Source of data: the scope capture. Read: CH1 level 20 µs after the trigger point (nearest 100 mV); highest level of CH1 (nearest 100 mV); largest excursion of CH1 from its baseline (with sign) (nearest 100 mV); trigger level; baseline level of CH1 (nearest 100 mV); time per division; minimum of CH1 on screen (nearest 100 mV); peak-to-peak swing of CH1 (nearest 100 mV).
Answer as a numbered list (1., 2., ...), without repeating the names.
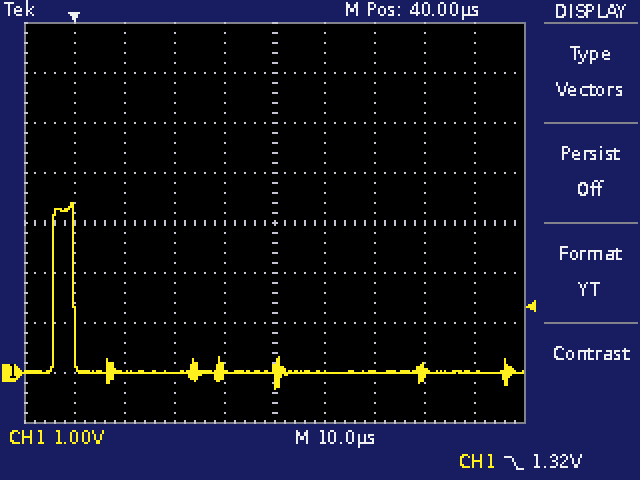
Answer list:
1. 0.0 V
2. 3.4 V
3. +3.4 V
4. 1.32 V
5. 0.0 V
6. 10 µs
7. -300 mV
8. 3.7 V
